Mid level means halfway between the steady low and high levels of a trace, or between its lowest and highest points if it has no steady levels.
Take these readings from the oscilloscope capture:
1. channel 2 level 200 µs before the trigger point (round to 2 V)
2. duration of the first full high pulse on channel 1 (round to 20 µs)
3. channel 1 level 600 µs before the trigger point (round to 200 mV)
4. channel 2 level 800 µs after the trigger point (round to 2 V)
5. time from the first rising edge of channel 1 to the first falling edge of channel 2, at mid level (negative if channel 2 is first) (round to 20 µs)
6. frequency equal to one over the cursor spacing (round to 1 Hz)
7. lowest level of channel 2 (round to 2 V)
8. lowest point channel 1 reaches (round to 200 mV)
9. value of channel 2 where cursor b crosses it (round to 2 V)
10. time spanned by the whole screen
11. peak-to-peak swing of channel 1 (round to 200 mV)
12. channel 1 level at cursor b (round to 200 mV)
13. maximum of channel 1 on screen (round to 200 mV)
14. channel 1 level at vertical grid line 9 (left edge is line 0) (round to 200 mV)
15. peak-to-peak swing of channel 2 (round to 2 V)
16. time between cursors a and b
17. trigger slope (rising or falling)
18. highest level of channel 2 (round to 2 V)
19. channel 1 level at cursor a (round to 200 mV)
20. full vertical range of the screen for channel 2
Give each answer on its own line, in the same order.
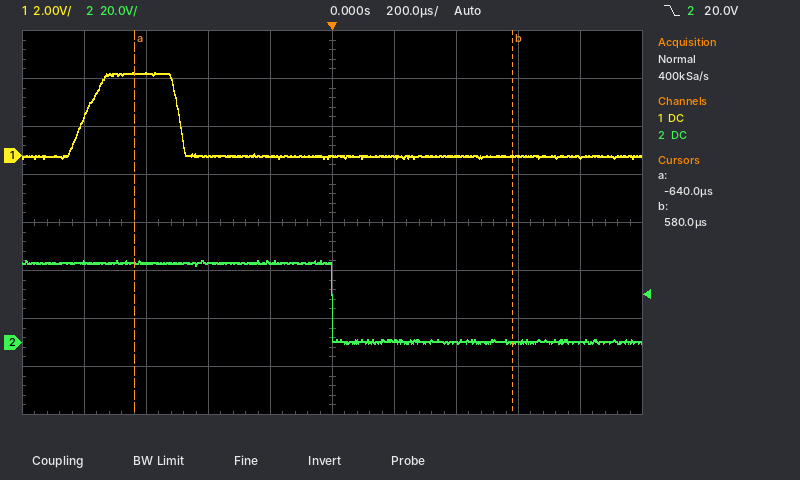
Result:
34 V
300 µs
3.4 V
0 V
+800 µs
820 Hz
0 V
-200 mV
0 V
2 ms
3.6 V
0.0 V
3.4 V
0.0 V
34 V
1.22 ms
falling
34 V
3.4 V
160 V
